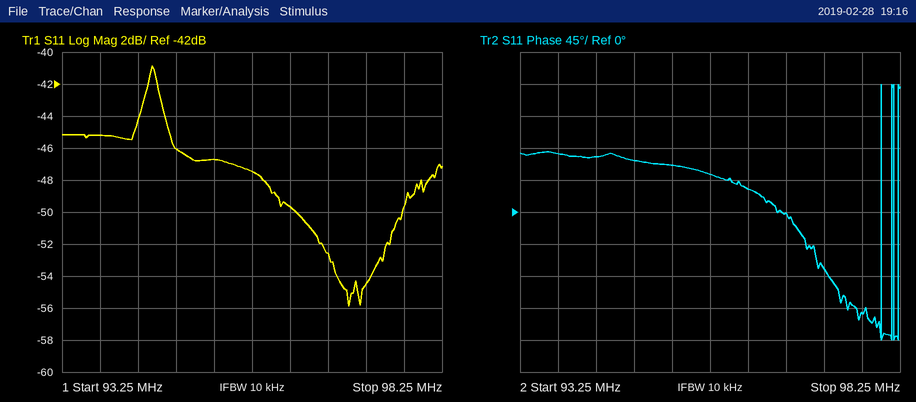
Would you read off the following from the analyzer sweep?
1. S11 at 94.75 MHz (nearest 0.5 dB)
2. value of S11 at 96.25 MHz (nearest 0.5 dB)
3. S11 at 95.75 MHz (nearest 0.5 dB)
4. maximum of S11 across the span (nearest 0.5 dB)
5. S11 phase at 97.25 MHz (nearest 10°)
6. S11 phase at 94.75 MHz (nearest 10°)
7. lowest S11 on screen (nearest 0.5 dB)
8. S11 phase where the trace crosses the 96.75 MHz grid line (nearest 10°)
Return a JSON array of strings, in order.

["-46.0 dB", "-49.5 dB", "-47.5 dB", "-41.0 dB", "-80°", "70°", "-56.0 dB", "0°"]
